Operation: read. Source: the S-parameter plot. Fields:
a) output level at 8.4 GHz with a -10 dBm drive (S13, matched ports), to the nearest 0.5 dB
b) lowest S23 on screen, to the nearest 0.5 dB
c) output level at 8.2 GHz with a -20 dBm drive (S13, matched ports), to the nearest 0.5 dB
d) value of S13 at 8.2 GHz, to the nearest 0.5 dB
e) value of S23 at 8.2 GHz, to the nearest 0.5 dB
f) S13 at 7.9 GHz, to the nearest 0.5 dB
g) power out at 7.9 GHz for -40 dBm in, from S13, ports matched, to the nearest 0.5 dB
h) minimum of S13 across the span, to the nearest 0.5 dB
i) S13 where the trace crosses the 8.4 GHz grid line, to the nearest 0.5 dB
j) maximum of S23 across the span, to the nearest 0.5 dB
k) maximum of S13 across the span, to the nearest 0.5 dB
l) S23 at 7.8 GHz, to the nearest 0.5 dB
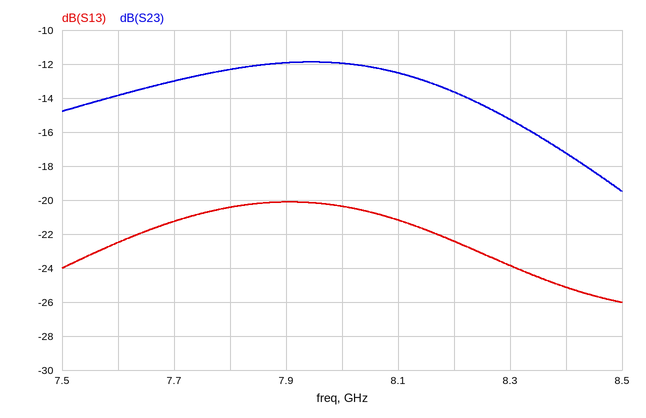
-35.0 dBm
-19.5 dB
-42.5 dBm
-22.5 dB
-13.5 dB
-20.0 dB
-60.0 dBm
-26.0 dB
-25.0 dB
-12.0 dB
-20.0 dB
-12.5 dB
